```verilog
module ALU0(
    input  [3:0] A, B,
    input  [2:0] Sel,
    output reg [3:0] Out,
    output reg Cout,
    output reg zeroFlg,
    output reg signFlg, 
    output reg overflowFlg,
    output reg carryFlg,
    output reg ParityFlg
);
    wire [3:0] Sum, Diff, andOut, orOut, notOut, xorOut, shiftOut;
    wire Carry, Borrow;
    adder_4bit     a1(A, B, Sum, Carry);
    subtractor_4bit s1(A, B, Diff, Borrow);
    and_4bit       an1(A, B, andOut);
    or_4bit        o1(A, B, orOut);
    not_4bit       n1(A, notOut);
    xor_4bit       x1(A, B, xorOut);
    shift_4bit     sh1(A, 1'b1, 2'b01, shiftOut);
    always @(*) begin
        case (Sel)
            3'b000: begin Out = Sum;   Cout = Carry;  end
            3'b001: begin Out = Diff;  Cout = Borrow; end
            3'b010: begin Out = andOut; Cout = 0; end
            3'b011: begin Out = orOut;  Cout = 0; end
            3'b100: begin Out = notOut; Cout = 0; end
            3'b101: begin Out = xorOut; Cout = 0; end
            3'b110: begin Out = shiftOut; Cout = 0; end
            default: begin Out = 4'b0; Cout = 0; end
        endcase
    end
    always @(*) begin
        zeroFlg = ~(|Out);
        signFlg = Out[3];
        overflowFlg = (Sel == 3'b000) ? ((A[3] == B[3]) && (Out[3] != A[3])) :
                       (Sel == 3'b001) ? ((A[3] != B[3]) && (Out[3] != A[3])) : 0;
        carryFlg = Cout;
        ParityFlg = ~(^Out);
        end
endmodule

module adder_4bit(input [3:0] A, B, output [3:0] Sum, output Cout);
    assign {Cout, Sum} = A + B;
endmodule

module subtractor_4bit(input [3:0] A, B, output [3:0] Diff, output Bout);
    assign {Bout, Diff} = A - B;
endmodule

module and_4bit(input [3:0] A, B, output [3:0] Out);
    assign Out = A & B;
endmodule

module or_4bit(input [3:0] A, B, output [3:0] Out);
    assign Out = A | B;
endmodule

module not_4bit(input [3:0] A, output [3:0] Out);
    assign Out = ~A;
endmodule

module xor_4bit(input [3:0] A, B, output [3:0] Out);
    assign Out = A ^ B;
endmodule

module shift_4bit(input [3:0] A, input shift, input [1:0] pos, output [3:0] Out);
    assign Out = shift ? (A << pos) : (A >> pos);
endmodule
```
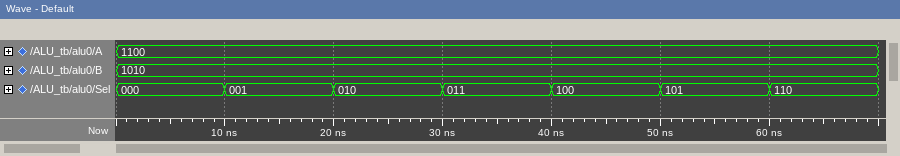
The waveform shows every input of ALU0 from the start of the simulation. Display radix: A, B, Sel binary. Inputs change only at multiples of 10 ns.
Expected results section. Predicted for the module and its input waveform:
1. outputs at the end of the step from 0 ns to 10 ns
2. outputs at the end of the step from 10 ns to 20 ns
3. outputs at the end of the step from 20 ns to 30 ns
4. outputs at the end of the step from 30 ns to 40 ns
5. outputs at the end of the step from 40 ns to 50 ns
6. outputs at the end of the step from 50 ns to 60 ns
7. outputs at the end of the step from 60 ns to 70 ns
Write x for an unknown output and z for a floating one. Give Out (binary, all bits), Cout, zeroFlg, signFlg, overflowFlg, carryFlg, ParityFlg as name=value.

Out=0110, Cout=1, zeroFlg=0, signFlg=0, overflowFlg=1, carryFlg=1, ParityFlg=1
Out=0010, Cout=0, zeroFlg=0, signFlg=0, overflowFlg=0, carryFlg=0, ParityFlg=0
Out=1000, Cout=0, zeroFlg=0, signFlg=1, overflowFlg=0, carryFlg=0, ParityFlg=0
Out=1110, Cout=0, zeroFlg=0, signFlg=1, overflowFlg=0, carryFlg=0, ParityFlg=0
Out=0011, Cout=0, zeroFlg=0, signFlg=0, overflowFlg=0, carryFlg=0, ParityFlg=1
Out=0110, Cout=0, zeroFlg=0, signFlg=0, overflowFlg=0, carryFlg=0, ParityFlg=1
Out=1000, Cout=0, zeroFlg=0, signFlg=1, overflowFlg=0, carryFlg=0, ParityFlg=0
